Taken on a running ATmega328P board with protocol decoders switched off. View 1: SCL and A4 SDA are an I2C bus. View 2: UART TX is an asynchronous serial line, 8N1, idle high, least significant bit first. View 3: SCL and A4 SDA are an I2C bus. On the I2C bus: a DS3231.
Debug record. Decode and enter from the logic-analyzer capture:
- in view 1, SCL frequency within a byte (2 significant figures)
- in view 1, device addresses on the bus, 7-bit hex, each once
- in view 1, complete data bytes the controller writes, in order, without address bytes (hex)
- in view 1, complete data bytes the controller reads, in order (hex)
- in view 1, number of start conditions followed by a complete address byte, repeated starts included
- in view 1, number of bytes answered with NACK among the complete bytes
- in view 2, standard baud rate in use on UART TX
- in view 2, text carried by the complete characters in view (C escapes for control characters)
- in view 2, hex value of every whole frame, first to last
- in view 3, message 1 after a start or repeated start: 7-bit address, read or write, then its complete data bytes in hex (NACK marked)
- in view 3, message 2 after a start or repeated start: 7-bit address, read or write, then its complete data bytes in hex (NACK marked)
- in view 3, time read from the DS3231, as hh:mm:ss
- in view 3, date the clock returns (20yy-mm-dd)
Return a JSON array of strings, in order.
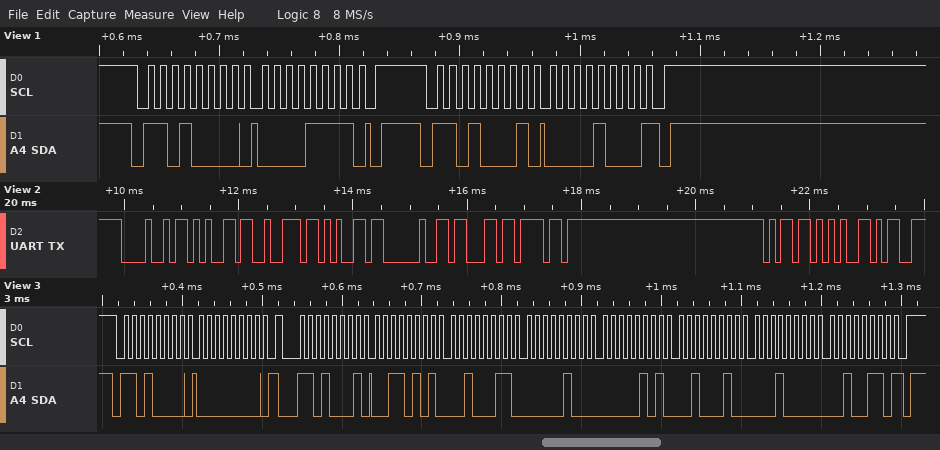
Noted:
["100 kHz", "0x68", "0F", "08", "2", "1", "9600 baud", "\"Here come\"", "48 65 72 65 20 63 6F 6D 65", "0x68 write: 00", "0x68 read: 35 23 04 05 22 10 26 NACK", "04:23:35", "2026-10-22"]
